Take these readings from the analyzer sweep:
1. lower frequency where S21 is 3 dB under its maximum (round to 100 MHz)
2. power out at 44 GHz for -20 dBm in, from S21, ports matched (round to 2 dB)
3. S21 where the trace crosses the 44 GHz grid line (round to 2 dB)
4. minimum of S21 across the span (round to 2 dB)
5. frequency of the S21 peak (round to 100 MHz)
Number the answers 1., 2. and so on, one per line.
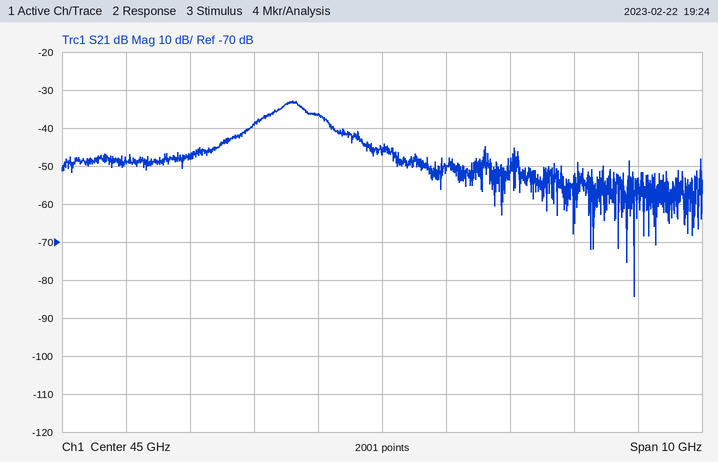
1. 43.3 GHz
2. -56 dBm
3. -36 dB
4. -84 dB
5. 43.6 GHz
